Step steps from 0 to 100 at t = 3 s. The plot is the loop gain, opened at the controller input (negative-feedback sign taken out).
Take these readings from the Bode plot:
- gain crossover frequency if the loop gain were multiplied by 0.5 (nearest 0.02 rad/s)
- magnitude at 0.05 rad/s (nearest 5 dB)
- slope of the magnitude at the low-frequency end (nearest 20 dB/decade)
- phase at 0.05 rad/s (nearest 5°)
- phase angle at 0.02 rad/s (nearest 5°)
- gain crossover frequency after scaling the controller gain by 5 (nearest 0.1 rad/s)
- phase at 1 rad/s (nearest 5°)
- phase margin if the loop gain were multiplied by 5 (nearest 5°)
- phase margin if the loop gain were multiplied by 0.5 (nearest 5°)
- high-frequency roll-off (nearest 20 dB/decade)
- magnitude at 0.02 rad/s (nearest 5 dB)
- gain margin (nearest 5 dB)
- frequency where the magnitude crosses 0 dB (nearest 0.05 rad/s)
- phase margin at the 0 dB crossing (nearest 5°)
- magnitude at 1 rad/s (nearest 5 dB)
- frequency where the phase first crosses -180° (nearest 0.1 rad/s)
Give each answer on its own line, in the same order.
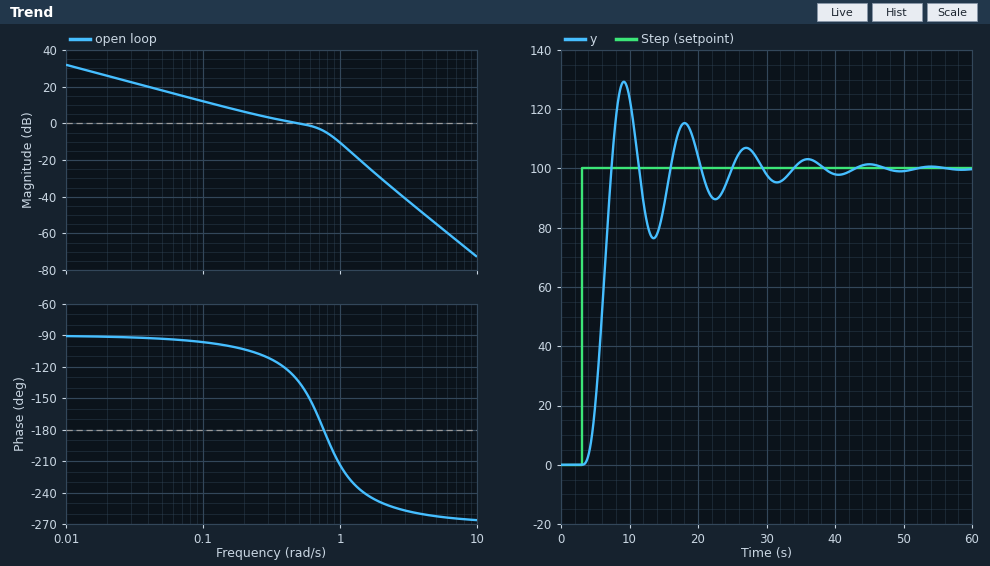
0.20 rad/s
20 dB
-20 dB/decade
-95°
-90°
1.1 rad/s
-215°
-45°
75°
-60 dB/decade
25 dB
5 dB
0.50 rad/s
45°
-10 dB
0.8 rad/s
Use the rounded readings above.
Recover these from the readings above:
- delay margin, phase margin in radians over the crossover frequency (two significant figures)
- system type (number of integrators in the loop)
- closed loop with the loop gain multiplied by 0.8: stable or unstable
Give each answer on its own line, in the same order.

1.6 s
1
stable
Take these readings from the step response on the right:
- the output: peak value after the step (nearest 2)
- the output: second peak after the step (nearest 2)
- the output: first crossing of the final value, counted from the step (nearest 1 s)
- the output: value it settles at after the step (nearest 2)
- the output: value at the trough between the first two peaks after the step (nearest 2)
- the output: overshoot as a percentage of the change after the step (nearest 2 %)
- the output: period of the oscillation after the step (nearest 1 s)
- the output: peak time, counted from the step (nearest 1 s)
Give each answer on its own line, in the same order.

130
116
4 s
100
76
30 %
9 s
6 s
